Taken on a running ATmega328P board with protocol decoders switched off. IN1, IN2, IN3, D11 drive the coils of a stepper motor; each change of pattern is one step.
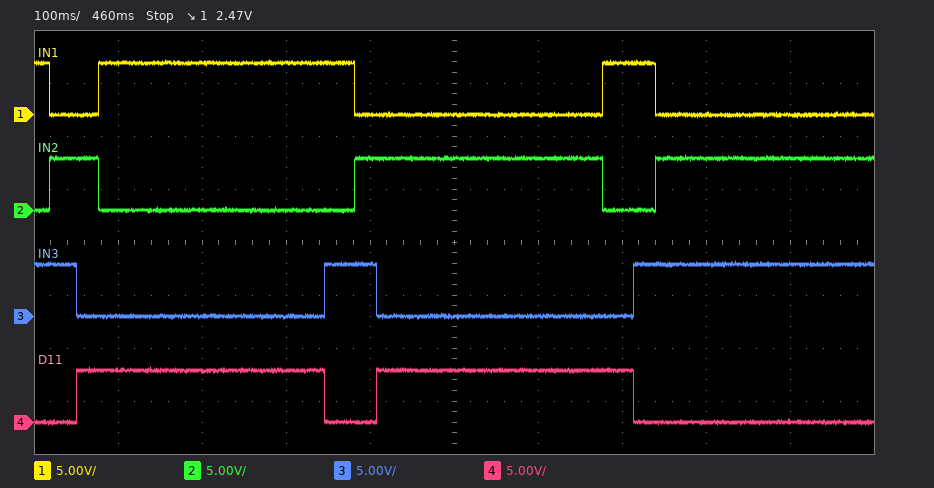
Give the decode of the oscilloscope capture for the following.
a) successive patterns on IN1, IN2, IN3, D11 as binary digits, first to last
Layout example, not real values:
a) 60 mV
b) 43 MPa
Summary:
a) 1010 0110 0101 1001 1010 0110 0101 1001 1010 0110
